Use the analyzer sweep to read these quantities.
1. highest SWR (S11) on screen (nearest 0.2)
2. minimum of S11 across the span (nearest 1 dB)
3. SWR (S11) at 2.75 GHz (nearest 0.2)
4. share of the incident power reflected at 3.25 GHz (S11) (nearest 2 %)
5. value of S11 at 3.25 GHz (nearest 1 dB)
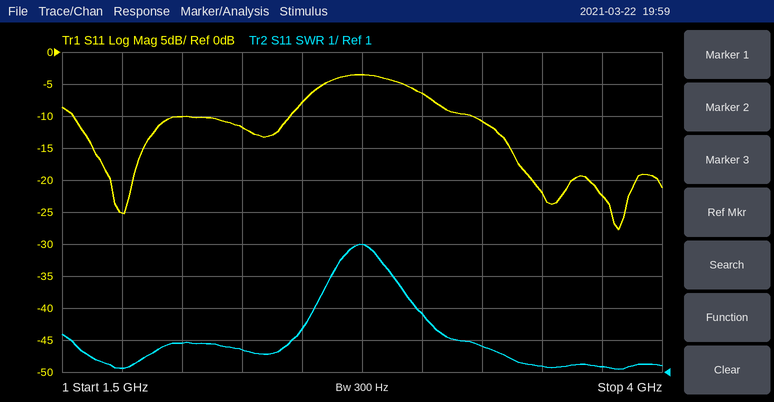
5.0
-28 dB
5.0
8 %
-11 dB
